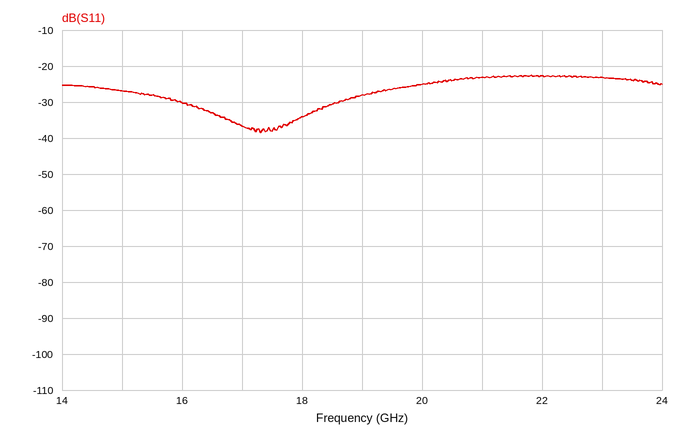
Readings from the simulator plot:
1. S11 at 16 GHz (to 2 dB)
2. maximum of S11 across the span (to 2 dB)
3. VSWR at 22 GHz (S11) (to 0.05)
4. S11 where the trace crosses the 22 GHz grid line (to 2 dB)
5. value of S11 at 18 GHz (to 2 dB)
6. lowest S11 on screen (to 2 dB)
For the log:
-30 dB
-22 dB
1.15
-22 dB
-34 dB
-38 dB
